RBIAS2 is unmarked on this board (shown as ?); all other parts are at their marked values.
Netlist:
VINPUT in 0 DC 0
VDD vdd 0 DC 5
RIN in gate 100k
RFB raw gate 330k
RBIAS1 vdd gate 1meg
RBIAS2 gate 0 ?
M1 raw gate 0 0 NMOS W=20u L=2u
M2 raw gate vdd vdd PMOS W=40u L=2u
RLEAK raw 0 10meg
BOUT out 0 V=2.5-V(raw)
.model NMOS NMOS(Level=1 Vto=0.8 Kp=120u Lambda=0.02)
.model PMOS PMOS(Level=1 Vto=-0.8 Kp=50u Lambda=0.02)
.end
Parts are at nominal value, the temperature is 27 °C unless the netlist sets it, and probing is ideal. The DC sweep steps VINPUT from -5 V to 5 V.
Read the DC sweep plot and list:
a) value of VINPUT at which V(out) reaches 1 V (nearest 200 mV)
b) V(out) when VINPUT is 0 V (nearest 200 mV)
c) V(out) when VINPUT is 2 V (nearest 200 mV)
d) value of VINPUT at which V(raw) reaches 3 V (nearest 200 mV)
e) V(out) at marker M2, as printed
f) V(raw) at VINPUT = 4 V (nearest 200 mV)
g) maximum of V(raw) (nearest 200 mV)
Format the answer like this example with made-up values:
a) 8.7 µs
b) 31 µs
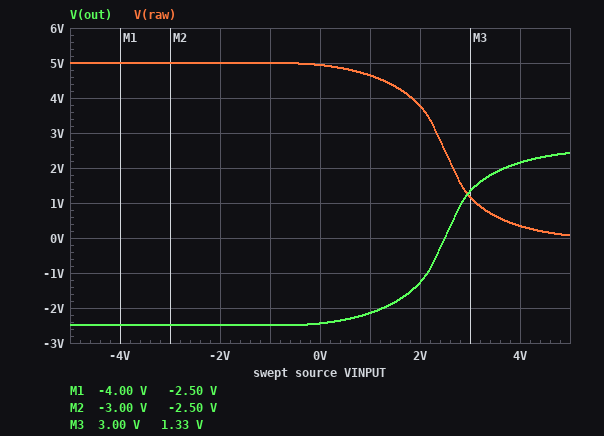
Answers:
a) 2.8 V
b) -2.4 V
c) -1.2 V
d) 2.4 V
e) -2.50 V
f) 400 mV
g) 5.0 V
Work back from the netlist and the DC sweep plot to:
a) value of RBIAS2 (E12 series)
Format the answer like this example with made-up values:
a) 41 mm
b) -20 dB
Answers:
a) 680 kΩ
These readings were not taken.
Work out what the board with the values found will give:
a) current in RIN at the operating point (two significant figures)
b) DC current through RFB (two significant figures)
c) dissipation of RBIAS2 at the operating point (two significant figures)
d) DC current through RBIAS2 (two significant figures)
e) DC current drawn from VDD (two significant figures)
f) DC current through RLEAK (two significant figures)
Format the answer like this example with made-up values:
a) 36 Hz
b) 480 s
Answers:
a) 13 µA
b) 11 µA
c) 2.4 µW
d) 1.9 µA
e) 170 µA
f) 490 nA
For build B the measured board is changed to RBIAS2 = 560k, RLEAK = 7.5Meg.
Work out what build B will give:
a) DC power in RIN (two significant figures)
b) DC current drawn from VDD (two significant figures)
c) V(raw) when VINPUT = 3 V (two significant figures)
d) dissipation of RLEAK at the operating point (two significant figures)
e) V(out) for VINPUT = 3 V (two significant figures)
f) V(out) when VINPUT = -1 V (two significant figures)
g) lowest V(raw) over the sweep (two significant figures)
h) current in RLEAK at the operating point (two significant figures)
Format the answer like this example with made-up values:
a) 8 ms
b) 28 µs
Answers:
a) 16 µW
b) 160 µA
c) 1.3 V
d) 3.3 µW
e) 1.2 V
f) -2.5 V
g) 89 mV
h) 660 nA
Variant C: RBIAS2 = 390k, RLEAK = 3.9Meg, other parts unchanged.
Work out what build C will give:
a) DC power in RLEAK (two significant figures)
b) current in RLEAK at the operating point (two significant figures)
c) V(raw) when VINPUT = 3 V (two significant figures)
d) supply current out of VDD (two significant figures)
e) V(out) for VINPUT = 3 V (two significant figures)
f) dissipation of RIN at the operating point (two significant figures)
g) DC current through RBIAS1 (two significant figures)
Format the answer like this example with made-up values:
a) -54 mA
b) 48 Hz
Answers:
a) 6.3 µW
b) 1.3 µA
c) 1.8 V
d) 130 µA
e) 720 mV
f) 15 µW
g) 3.8 µA
